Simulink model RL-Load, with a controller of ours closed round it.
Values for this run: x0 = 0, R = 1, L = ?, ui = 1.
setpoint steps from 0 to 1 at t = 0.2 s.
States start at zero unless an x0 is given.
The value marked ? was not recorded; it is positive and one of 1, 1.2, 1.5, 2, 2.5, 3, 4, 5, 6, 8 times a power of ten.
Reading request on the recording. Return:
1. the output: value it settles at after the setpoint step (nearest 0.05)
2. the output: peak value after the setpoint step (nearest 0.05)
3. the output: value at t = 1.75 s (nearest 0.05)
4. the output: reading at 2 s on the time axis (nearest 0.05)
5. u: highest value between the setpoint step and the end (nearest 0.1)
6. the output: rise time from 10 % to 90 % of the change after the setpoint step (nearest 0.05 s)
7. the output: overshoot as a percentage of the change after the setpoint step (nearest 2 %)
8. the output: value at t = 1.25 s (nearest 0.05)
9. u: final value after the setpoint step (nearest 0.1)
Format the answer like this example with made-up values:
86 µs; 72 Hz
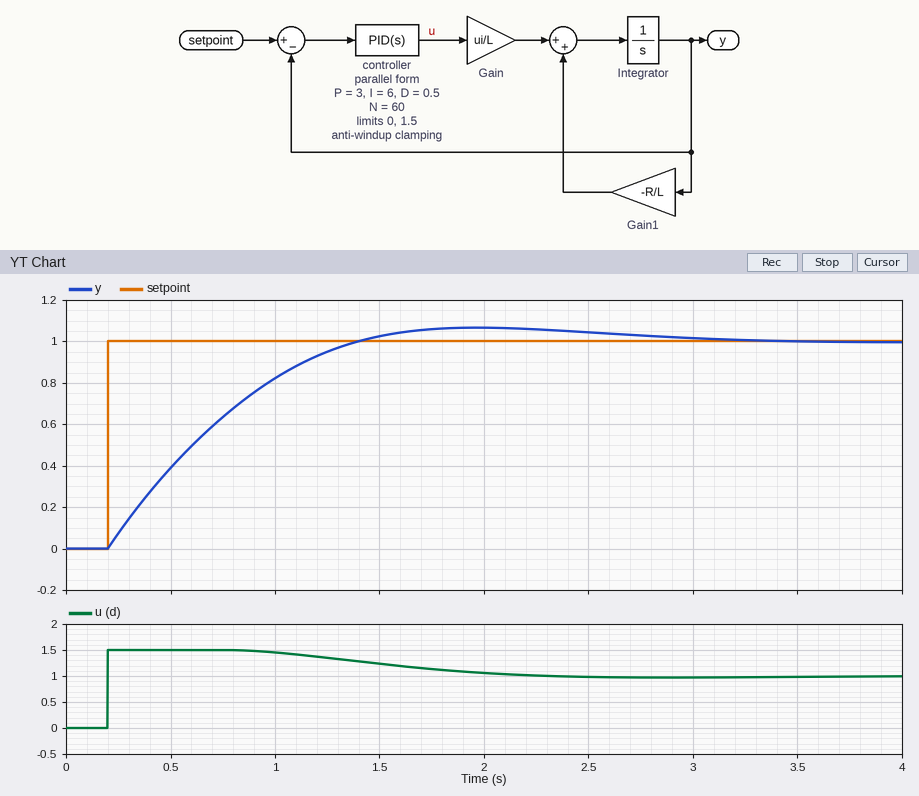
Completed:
1.00; 1.05; 1.05; 1.05; 1.5; 0.85 s; 6 %; 0.95; 1.0
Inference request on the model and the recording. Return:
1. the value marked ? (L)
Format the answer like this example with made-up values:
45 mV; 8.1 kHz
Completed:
1
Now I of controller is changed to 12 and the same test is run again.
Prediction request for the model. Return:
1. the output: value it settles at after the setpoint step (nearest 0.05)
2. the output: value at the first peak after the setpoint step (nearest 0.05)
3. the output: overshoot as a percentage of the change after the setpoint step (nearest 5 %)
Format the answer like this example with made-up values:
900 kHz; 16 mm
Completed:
1.00; 1.10; 10 %
